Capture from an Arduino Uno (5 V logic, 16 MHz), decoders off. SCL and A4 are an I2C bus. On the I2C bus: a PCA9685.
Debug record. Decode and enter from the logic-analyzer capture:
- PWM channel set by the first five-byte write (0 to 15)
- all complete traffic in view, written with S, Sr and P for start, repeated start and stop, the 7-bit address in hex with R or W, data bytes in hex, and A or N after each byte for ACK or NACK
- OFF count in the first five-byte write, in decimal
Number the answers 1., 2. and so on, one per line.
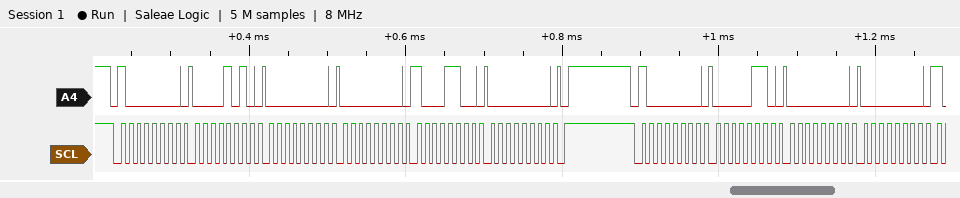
1. 1
2. S 40W A 0A A 00 A 00 A 8C A 00 A P S 40W A 06 A 00 A 00 A
3. 140
